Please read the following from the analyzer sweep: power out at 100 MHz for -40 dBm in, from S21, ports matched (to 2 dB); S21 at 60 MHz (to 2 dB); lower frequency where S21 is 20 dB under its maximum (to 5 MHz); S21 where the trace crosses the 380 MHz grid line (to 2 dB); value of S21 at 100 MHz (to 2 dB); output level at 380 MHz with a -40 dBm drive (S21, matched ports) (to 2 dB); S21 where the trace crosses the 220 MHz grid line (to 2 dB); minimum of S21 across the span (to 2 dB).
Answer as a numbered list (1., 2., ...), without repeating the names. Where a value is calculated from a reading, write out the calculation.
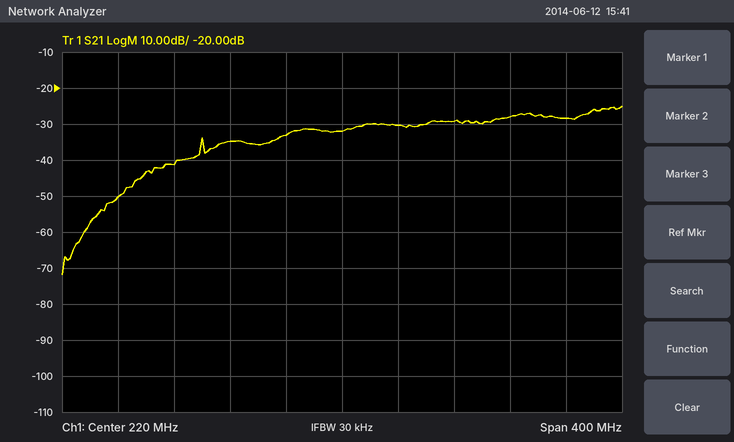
1. -40 dBm + (-42 dB) = -82 dBm
2. -50 dB
3. 75 MHz
4. -28 dB
5. -42 dB
6. -40 dBm + (-28 dB) = -68 dBm
7. -32 dB
8. -72 dB
